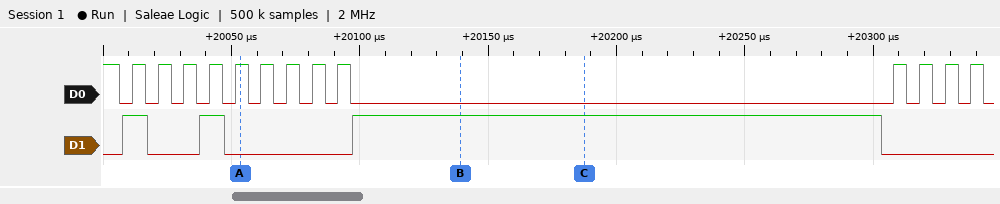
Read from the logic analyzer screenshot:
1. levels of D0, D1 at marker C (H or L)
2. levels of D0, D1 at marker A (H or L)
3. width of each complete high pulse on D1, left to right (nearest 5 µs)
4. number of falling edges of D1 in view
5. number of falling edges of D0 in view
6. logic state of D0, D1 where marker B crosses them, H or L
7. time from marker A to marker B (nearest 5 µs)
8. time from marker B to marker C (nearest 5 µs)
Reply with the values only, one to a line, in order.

D0=L, D1=H
D0=H, D1=L
10 µs, 10 µs, 205 µs
3
14
D0=L, D1=H
85 µs
50 µs
